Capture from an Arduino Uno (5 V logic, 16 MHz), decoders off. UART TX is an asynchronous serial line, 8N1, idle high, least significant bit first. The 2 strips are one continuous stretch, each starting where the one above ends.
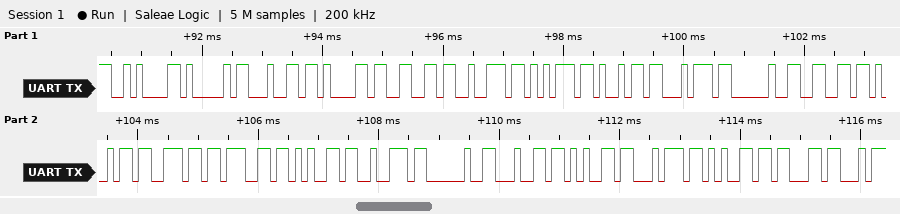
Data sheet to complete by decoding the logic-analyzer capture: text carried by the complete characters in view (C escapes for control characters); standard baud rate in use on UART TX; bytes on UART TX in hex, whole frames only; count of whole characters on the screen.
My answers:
"\nAdafruit finger detec"
9600 baud
0A 41 64 61 66 72 75 69 74 20 66 69 6E 67 65 72 20 64 65 74 65 63
22
